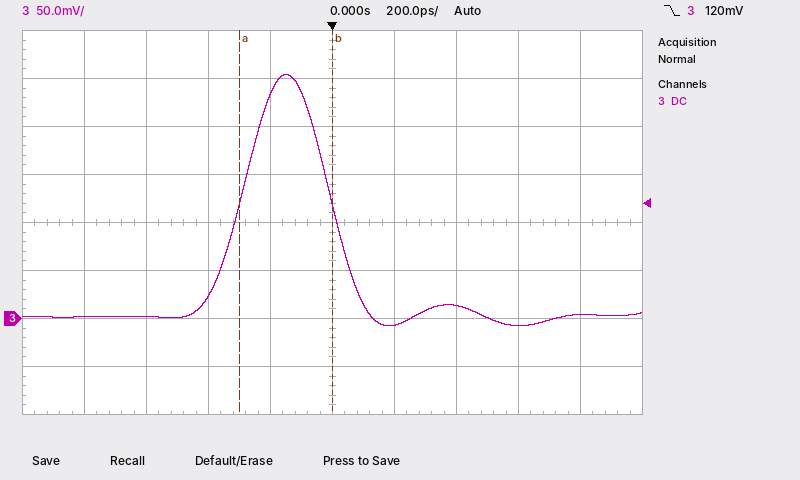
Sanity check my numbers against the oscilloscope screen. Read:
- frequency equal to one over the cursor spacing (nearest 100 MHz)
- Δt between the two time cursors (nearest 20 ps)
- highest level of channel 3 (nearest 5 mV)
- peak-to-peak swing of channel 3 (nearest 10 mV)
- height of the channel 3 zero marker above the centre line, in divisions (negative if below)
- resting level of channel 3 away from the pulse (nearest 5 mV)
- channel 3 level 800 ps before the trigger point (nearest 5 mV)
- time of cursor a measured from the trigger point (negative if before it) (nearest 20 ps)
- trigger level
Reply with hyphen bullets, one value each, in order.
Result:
- 3.3 GHz
- 300 ps
- 255 mV
- 260 mV
- -2.0 div
- 0 mV
- 0 mV
- -300 ps
- 120 mV
